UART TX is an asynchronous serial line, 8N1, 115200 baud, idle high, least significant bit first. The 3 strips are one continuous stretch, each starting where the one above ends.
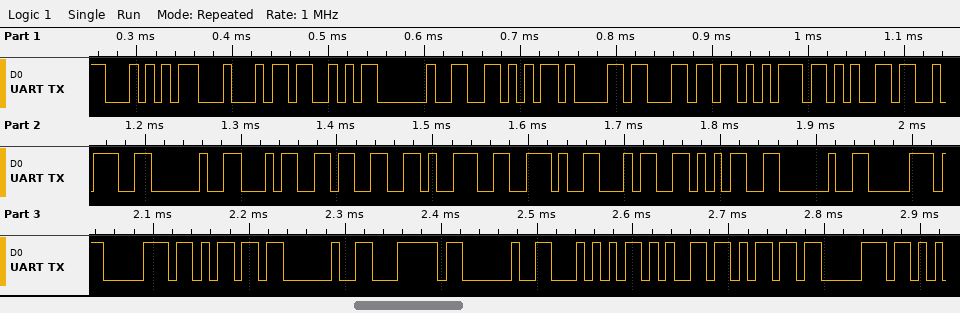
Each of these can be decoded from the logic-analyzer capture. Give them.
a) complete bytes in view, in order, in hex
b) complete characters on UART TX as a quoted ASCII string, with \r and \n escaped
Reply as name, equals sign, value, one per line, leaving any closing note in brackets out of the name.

complete bytes in view, in order, in hex = 54 44 53 20 56 61 6C 75 65 3A 20 34 33 39 2E 34 35 20 70 70 6D 20 7C 20 54 65 6D 70
complete characters on UART TX as a quoted ASCII string, with \r and \n escaped = "TDS Value: 439.45 ppm | Temp"
